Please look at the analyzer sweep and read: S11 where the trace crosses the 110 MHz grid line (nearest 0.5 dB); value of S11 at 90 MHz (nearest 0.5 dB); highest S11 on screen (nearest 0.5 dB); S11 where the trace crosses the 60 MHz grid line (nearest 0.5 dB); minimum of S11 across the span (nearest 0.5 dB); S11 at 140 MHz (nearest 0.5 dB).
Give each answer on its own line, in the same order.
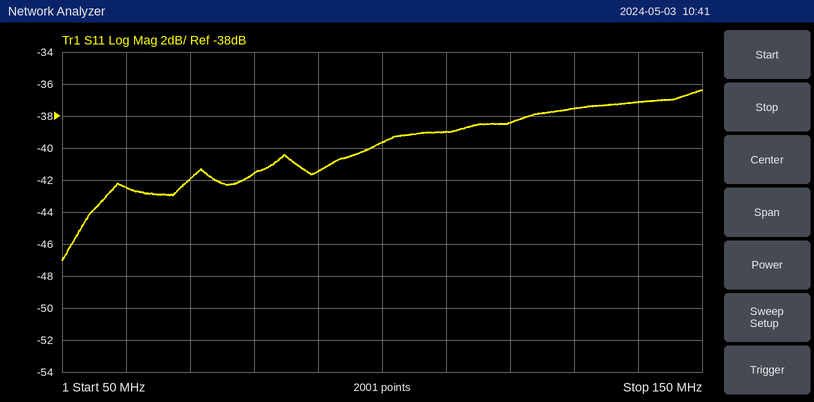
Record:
-39.0 dB
-41.5 dB
-36.5 dB
-42.5 dB
-47.0 dB
-37.0 dB
